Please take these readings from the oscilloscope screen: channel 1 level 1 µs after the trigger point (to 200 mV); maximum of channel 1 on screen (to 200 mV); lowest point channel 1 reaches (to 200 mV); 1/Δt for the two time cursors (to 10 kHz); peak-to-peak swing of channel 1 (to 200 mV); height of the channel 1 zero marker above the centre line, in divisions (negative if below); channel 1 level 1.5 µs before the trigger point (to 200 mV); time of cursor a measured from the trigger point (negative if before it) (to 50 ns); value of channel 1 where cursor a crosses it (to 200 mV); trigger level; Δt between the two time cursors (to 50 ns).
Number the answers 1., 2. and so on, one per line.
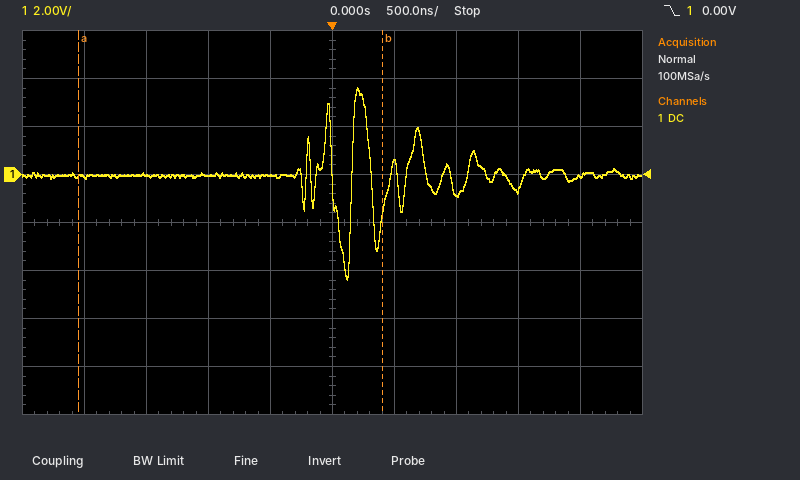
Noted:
1. -800 mV
2. 3.6 V
3. -4.4 V
4. 410 kHz
5. 8.0 V
6. +1.0 div
7. 0.0 V
8. -2.05 µs
9. 0.0 V
10. 0.00 V
11. 2.45 µs
